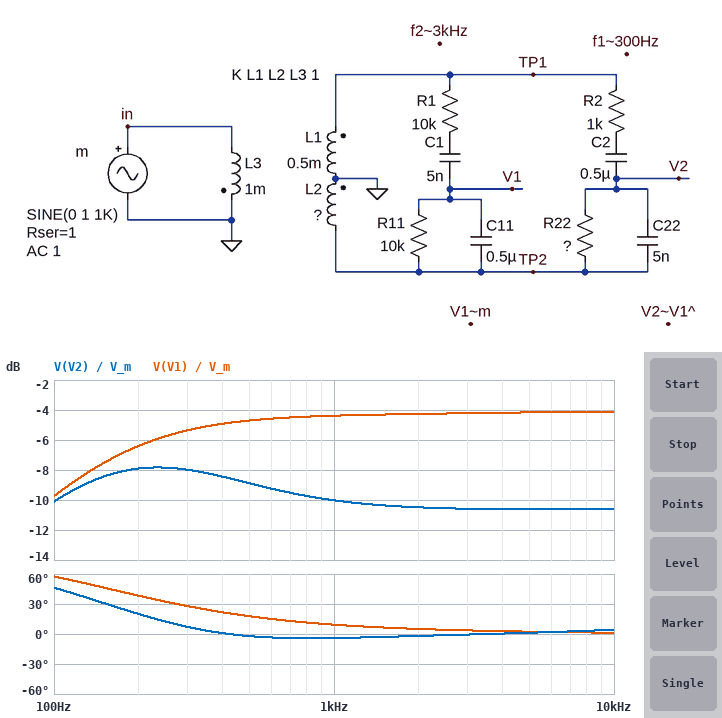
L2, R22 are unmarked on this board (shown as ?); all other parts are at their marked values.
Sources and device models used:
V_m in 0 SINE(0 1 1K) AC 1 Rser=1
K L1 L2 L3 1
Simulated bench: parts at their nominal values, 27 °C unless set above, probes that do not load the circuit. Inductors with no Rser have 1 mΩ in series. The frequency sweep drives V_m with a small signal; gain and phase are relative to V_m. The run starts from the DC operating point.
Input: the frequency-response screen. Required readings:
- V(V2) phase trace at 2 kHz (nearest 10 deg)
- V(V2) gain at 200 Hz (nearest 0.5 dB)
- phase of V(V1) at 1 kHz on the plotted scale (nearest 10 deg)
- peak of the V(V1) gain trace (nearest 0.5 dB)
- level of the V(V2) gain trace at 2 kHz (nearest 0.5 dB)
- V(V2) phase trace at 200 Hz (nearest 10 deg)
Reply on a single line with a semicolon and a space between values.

0 deg; -8.0 dB; 10 deg; -4.0 dB; -10.5 dB; 20 deg
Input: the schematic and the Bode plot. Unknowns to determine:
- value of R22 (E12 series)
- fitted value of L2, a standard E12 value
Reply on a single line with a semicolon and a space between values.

330 Ω; 390 µH
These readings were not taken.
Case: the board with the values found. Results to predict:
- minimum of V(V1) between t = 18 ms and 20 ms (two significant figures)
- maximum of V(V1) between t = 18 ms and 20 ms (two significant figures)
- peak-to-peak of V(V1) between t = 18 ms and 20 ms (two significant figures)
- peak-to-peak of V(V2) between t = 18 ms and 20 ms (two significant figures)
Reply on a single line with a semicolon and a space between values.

-600 mV; 600 mV; 1.2 V; 630 mV
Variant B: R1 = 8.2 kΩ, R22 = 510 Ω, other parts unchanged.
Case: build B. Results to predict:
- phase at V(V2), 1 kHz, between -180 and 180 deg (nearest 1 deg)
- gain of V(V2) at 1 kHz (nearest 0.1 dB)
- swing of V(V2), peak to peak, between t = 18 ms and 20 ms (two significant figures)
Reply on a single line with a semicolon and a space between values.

-15 deg; -13.6 dB; 420 mV
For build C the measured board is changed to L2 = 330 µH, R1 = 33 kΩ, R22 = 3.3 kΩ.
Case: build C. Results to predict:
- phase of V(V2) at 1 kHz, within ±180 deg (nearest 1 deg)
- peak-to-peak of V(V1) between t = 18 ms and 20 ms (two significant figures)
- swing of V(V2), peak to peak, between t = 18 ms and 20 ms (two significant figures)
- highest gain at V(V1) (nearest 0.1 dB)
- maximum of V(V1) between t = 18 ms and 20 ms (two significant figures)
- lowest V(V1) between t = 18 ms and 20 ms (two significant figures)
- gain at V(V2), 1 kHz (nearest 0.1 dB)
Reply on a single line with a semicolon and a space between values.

-164 deg; 1.1 V; 790 mV; -4.8 dB; 560 mV; -560 mV; -8.0 dB
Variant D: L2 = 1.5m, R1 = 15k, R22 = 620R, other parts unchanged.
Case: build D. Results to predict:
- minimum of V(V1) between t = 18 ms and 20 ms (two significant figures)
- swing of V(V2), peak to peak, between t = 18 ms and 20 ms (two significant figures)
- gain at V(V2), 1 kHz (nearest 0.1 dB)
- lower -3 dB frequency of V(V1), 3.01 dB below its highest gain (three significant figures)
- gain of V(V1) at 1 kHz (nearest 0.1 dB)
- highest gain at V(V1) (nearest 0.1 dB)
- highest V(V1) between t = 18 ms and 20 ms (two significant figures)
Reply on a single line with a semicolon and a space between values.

-1.2 V; 1.0 V; -5.7 dB; 163 Hz; 1.5 dB; 1.7 dB; 1.2 V
